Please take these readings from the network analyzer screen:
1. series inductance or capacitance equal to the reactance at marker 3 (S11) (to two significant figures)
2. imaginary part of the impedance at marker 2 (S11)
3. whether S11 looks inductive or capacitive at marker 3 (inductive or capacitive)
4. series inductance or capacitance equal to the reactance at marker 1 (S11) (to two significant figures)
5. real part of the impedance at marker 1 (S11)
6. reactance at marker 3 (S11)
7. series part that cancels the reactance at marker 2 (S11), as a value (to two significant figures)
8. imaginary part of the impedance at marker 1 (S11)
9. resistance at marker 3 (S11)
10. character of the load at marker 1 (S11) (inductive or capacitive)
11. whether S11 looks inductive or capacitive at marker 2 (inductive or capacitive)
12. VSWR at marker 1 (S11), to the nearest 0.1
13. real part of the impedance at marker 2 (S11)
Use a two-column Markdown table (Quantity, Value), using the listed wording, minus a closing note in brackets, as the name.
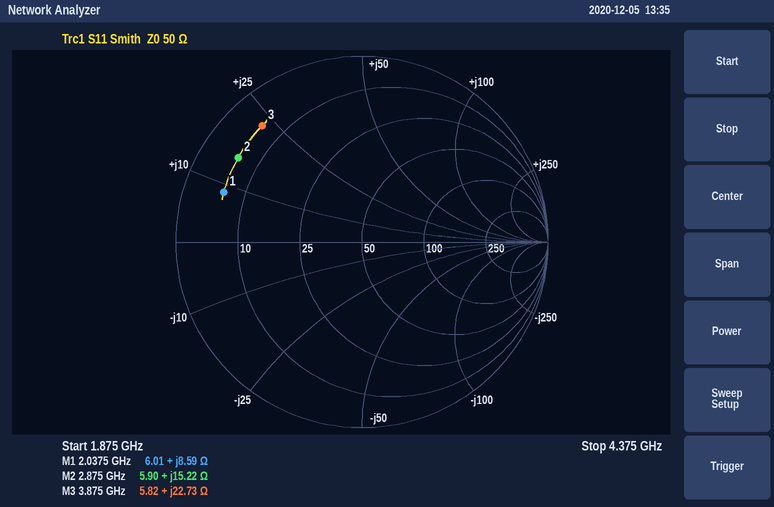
| Quantity | Value |
|---|---|
| series inductance or capacitance equal to the reactance at marker 3 (S11) | 930 pH |
| imaginary part of the impedance at marker 2 | +15.22 Ω |
| whether S11 looks inductive or capacitive at marker 3 | inductive |
| series inductance or capacitance equal to the reactance at marker 1 (S11) | 670 pH |
| real part of the impedance at marker 1 | 6.01 Ω |
| reactance at marker 3 | +22.73 Ω |
| series part that cancels the reactance at marker 2 (S11), as a value | 3.6 pF |
| imaginary part of the impedance at marker 1 | +8.59 Ω |
| resistance at marker 3 | 5.82 Ω |
| character of the load at marker 1 (S11) | inductive |
| whether S11 looks inductive or capacitive at marker 2 | inductive |
| VSWR at marker 1 (S11), to the nearest 0.1 | 8.6 |
| real part of the impedance at marker 2 | 5.90 Ω |
